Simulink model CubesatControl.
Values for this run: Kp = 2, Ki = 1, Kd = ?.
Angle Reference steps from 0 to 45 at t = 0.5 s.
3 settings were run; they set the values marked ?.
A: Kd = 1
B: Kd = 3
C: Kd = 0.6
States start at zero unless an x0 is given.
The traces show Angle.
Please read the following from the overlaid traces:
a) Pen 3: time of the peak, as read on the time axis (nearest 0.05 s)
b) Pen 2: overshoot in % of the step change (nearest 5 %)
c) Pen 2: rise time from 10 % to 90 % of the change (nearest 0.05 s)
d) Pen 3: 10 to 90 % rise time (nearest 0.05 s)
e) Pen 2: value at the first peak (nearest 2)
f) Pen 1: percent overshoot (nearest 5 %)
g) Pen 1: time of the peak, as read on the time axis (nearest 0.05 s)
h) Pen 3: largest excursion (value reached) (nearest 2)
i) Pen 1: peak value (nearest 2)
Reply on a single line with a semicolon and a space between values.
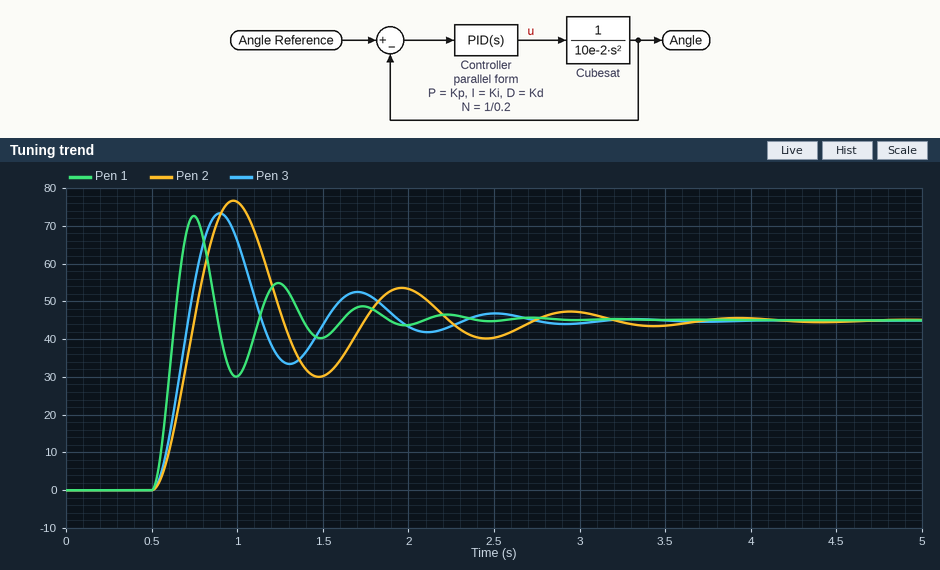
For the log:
0.90 s; 70 %; 0.15 s; 0.15 s; 76; 60 %; 0.75 s; 74; 72
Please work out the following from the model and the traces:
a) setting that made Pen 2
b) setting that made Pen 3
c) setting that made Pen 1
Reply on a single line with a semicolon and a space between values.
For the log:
C; A; B
